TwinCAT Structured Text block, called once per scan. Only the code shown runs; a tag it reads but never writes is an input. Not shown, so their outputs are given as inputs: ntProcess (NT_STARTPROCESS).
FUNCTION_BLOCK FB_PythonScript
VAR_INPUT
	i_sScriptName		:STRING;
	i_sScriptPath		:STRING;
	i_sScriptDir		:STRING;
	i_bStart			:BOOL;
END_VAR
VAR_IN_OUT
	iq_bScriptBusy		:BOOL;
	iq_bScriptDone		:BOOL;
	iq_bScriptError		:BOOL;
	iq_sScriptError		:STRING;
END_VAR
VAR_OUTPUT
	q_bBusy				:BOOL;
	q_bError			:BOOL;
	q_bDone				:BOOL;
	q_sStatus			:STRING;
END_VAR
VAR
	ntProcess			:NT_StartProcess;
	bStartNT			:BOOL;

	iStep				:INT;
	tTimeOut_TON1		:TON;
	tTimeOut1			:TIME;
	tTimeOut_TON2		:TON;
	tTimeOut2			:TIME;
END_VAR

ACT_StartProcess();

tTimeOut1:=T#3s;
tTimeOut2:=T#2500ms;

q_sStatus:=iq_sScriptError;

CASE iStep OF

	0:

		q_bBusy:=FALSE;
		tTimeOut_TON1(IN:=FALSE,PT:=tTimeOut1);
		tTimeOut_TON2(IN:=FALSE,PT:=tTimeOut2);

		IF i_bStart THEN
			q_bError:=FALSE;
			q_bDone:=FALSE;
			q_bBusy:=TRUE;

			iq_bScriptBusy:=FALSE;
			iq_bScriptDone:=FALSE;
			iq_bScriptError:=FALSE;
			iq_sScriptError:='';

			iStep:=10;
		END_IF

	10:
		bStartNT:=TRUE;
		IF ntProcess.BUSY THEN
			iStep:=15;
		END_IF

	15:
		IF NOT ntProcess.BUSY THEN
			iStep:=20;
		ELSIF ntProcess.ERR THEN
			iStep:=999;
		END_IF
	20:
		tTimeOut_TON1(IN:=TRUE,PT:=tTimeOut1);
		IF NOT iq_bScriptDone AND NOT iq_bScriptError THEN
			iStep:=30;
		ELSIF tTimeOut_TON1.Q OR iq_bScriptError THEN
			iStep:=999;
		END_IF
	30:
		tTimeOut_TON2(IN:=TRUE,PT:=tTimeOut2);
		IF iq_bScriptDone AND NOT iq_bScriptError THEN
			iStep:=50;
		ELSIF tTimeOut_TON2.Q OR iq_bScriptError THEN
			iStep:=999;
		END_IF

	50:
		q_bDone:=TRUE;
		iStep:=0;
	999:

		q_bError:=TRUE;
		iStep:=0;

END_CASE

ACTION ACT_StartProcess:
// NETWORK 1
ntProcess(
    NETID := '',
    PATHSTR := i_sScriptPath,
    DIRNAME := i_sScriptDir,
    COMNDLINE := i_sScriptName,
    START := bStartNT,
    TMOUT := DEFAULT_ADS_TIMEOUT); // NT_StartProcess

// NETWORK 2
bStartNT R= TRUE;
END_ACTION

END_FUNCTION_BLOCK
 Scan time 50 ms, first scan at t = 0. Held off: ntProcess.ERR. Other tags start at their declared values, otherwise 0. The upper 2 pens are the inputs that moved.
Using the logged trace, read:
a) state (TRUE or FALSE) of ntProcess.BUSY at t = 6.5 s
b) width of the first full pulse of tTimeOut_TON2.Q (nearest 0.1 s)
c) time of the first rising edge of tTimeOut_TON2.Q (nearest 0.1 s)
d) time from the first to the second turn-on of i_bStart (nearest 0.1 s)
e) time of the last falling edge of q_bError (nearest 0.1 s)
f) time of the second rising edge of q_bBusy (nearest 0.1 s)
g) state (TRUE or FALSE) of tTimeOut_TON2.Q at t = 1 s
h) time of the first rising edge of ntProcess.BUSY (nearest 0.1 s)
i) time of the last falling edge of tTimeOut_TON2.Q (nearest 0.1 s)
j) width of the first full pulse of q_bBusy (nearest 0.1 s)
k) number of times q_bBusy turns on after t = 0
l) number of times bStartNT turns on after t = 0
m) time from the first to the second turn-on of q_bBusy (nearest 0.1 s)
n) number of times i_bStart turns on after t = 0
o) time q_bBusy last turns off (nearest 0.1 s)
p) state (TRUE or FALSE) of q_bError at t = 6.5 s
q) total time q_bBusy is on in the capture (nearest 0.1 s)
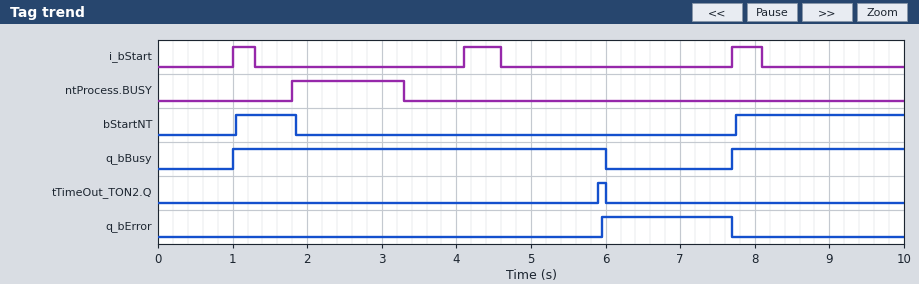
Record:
FALSE
0.1 s
5.9 s
3.1 s
7.7 s
7.7 s
FALSE
1.8 s
6.0 s
5.0 s
2
2
6.7 s
3
6.0 s
TRUE
7.3 s
